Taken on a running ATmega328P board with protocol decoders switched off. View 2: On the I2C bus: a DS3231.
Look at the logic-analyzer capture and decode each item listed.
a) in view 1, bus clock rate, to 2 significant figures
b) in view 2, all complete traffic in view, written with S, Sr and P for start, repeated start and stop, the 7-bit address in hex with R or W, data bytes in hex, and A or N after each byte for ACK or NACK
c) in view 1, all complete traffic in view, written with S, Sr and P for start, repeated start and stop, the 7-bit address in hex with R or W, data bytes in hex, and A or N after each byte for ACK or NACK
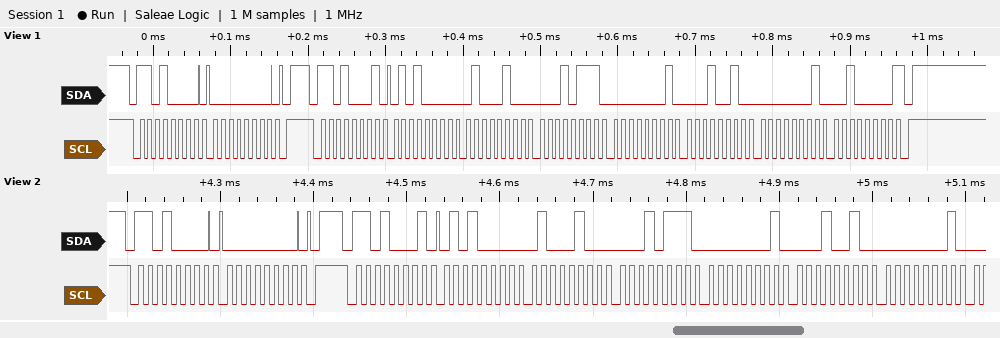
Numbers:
100 kHz
S 68W A 00 A P S 68R A 50 A 44 A 17 A 01 A 12 A 01 A
S 68W A 00 A P S 68R A 50 A 44 A 17 A 01 A 12 A 01 A 20 N P
